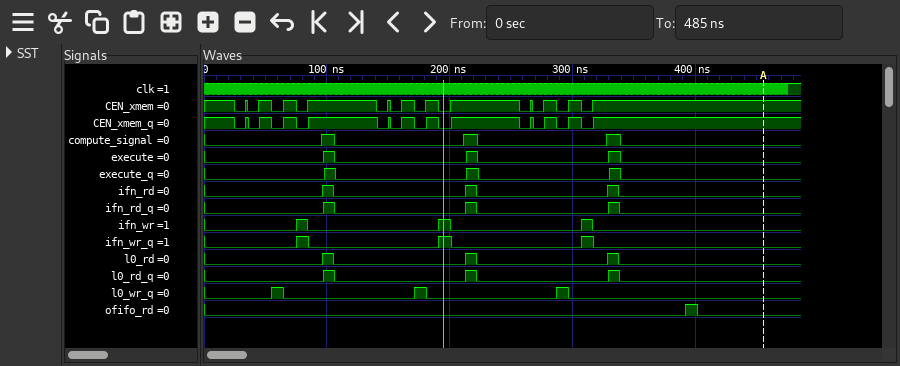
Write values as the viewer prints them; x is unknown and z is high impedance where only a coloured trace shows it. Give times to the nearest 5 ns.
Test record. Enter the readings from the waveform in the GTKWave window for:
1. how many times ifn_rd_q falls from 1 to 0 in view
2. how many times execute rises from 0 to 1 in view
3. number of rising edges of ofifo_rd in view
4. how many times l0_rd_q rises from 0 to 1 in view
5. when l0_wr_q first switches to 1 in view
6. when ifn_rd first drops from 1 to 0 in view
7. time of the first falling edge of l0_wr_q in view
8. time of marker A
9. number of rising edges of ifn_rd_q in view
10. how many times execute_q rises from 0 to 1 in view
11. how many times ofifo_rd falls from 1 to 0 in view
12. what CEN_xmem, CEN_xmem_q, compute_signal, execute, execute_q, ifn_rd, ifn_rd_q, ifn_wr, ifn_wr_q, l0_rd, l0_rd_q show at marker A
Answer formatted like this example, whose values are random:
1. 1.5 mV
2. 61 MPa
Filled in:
1. 3
2. 3
3. 1
4. 3
5. 55 ns
6. 105 ns
7. 65 ns
8. 455 ns
9. 3
10. 3
11. 1
12. CEN_xmem=1, CEN_xmem_q=1, compute_signal=0, execute=0, execute_q=0, ifn_rd=0, ifn_rd_q=0, ifn_wr=0, ifn_wr_q=0, l0_rd=0, l0_rd_q=0
